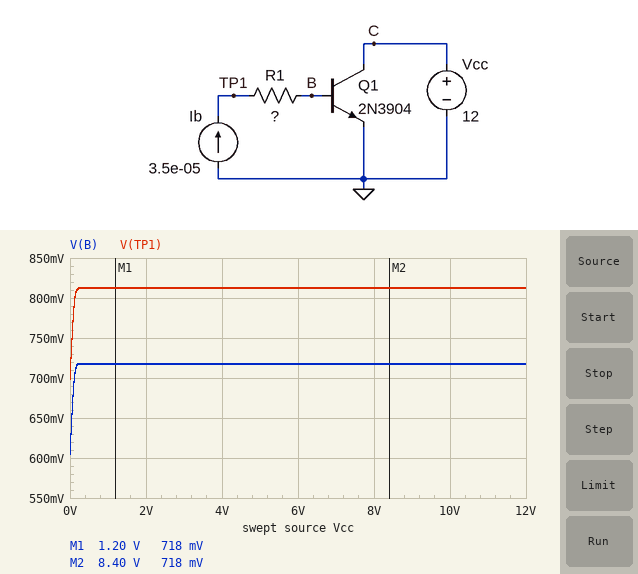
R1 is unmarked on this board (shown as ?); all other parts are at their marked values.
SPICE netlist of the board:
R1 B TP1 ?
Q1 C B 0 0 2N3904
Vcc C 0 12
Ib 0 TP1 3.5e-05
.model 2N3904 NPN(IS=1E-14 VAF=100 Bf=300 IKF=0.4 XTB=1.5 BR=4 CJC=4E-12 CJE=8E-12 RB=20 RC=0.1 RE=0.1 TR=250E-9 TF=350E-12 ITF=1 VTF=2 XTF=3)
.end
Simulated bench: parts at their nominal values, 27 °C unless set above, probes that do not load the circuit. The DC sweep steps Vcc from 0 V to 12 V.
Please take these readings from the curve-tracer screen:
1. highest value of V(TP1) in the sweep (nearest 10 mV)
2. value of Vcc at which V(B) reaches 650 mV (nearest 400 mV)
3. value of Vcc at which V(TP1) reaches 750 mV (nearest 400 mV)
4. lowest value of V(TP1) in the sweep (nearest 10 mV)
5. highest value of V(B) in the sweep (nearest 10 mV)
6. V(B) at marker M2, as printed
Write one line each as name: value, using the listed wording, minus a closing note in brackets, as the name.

highest value of V(TP1) in the sweep: 810 mV
value of Vcc at which V(B) reaches 650 mV: 0 V
value of Vcc at which V(TP1) reaches 750 mV: 0 V
lowest value of V(TP1) in the sweep: 700 mV
highest value of V(B) in the sweep: 720 mV
V(B) at marker M2, as printed: 718 mV
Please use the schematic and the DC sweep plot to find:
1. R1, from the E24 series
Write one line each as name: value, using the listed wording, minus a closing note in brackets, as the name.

R1, from the E24 series: 2.7 kΩ
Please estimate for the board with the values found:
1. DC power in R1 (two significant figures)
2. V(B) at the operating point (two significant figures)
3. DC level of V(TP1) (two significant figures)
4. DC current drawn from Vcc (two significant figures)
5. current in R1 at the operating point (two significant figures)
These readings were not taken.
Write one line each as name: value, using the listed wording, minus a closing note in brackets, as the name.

DC power in R1: 3.3 µW
V(B) at the operating point: 720 mV
DC level of V(TP1): 810 mV
DC current drawn from Vcc: 11 mA
current in R1 at the operating point: 35 µA
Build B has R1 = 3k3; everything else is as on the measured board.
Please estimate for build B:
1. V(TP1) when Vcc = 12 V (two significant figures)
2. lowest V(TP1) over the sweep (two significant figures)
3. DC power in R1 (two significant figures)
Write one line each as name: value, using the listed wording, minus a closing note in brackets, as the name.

V(TP1) when Vcc = 12 V: 830 mV
lowest V(TP1) over the sweep: 720 mV
DC power in R1: 4.0 µW
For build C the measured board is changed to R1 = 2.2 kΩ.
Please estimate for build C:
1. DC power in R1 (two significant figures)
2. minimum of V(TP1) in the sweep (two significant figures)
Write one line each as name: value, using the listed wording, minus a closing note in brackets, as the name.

DC power in R1: 2.7 µW
minimum of V(TP1) in the sweep: 680 mV
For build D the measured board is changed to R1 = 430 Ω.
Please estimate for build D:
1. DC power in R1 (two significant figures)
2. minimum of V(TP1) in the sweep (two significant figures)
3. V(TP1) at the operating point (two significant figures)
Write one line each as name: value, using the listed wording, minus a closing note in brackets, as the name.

DC power in R1: 530 nW
minimum of V(TP1) in the sweep: 620 mV
V(TP1) at the operating point: 730 mV
